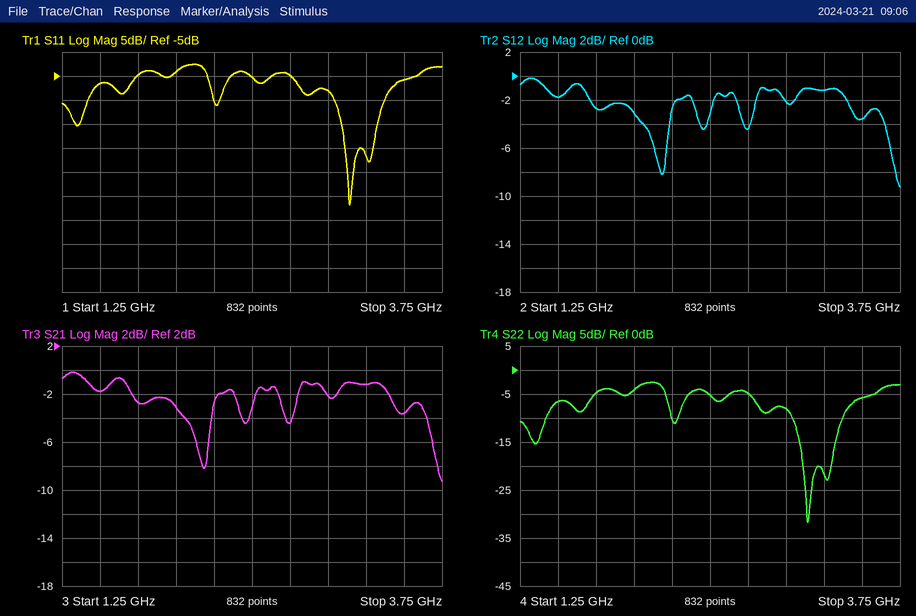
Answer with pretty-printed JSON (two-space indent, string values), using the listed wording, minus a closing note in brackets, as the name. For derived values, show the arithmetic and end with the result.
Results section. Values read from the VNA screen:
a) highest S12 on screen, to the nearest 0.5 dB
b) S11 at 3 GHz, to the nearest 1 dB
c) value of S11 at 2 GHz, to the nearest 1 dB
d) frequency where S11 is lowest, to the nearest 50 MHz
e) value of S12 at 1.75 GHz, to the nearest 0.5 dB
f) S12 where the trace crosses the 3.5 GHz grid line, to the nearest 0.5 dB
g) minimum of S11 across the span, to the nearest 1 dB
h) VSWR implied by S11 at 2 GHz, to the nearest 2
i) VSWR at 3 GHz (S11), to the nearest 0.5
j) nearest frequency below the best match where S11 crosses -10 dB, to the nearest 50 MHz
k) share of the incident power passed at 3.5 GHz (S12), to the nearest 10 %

{
  "highest S12 on screen, to the nearest 0.5 dB": "0.0 dB",
  "S11 at 3 GHz, to the nearest 1 dB": "-8 dB",
  "value of S11 at 2 GHz, to the nearest 1 dB": "-4 dB",
  "frequency where S11 is lowest, to the nearest 50 MHz": "3.15 GHz",
  "value of S12 at 1.75 GHz, to the nearest 0.5 dB": "-2.5 dB",
  "S12 where the trace crosses the 3.5 GHz grid line, to the nearest 0.5 dB": "-3.5 dB",
  "minimum of S11 across the span, to the nearest 1 dB": "-32 dB",
  "VSWR implied by S11 at 2 GHz, to the nearest 2": "|Γ| = 10^(-4/20) = 0.6310; VSWR = (1 + 0.6310)/(1 − 0.6310) ≈ 4",
  "VSWR at 3 GHz (S11), to the nearest 0.5": "|Γ| = 10^(-8/20) = 0.3981; VSWR = (1 + 0.3981)/(1 − 0.3981) ≈ 2.32, so 2.5 to the nearest 0.5",
  "nearest frequency below the best match where S11 crosses -10 dB, to the nearest 50 MHz": "3.05 GHz",
  "share of the incident power passed at 3.5 GHz (S12), to the nearest 10 %": "10^(-3.5/10) ≈ 44.7 %, so 40 % to the nearest 10 %"
}
